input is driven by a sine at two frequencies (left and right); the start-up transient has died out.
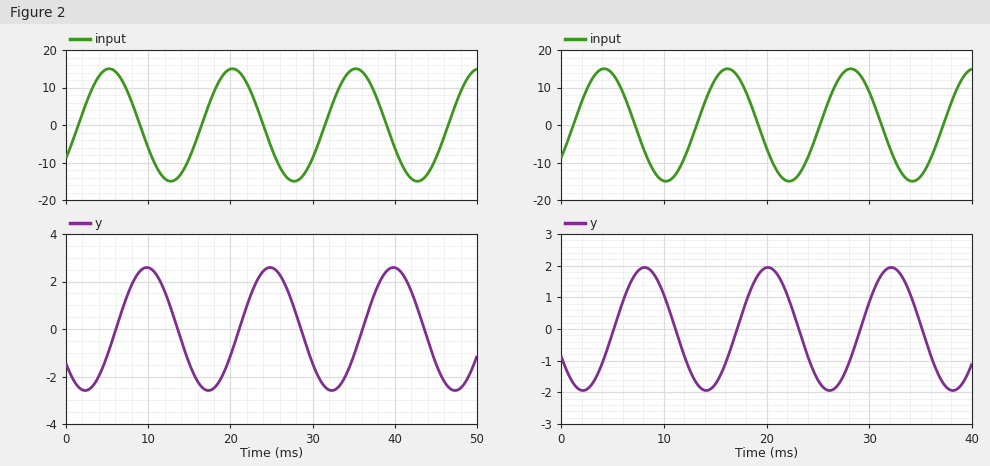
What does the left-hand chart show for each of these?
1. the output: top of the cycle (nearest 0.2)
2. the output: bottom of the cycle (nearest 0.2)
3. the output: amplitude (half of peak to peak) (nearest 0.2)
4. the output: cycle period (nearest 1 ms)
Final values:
2.6
-2.6
2.6
15 ms
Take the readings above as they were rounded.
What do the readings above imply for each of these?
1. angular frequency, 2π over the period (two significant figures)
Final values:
0.42 rad/ms
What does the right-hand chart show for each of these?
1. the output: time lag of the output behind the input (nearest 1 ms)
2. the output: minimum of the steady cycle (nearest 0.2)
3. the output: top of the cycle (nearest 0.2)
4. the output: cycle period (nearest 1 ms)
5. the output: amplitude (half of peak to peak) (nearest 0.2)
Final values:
4 ms
-2.0
2.0
12 ms
2.0
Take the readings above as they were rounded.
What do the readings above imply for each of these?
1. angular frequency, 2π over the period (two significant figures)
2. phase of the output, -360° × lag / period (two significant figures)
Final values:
0.52 rad/ms
-120°
